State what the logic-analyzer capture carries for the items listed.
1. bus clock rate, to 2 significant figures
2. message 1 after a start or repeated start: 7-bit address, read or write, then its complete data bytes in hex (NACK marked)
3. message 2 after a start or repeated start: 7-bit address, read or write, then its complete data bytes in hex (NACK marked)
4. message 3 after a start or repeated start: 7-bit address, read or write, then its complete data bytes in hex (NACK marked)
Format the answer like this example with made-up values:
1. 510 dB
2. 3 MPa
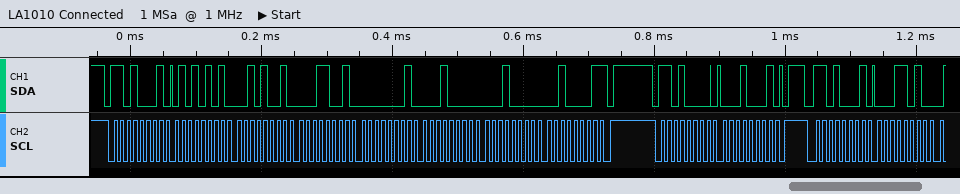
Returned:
1. 100 kHz
2. 0x68 read: 55 29 19 01 10 10 21 NACK
3. 0x68 write: 11
4. 0x68 read: 1A
